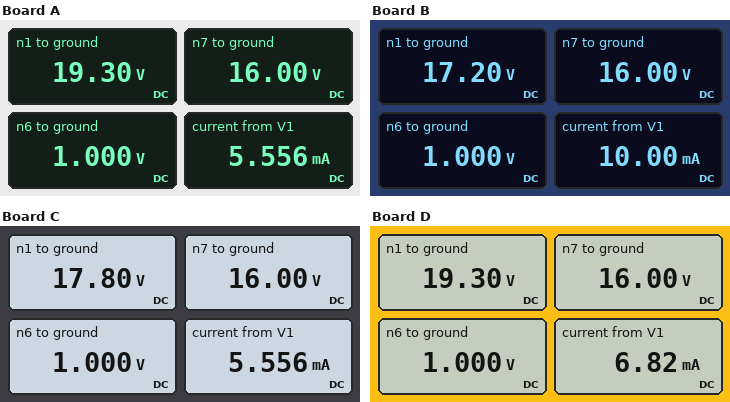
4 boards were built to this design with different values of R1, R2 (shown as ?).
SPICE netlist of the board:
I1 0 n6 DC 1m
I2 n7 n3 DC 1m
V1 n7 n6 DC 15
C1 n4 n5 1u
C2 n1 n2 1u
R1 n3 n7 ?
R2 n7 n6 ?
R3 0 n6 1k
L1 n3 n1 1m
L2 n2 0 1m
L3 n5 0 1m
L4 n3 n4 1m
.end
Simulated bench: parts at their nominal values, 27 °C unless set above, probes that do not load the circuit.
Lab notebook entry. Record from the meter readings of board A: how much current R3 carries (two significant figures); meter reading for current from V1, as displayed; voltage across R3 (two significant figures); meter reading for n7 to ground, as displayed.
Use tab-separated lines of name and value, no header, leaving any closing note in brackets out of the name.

how much current R3 carries	1.0 mA
meter reading for current from V1, as displayed	5.556 mA
voltage across R3	1.0 V
meter reading for n7 to ground, as displayed	16.00 V
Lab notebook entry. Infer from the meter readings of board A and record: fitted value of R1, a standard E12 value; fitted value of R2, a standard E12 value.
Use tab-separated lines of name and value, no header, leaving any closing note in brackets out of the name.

fitted value of R1, a standard E12 value	3.3 kΩ
fitted value of R2, a standard E12 value	2.7 kΩ
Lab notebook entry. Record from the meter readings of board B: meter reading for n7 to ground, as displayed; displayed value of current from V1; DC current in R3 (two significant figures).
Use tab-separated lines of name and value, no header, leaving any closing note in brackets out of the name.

meter reading for n7 to ground, as displayed	16.00 V
displayed value of current from V1	10.00 mA
DC current in R3	1.0 mA
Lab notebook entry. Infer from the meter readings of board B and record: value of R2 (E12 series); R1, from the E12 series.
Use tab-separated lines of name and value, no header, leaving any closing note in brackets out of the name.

value of R2	1.5 kΩ
R1, from the E12 series	1.2 kΩ
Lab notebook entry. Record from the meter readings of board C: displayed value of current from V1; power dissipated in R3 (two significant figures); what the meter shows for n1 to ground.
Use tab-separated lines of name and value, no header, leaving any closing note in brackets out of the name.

displayed value of current from V1	5.556 mA
power dissipated in R3	1.0 mW
what the meter shows for n1 to ground	17.80 V
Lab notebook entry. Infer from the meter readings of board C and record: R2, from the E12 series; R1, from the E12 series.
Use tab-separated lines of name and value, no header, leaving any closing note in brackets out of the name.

R2, from the E12 series	2.7 kΩ
R1, from the E12 series	1.8 kΩ
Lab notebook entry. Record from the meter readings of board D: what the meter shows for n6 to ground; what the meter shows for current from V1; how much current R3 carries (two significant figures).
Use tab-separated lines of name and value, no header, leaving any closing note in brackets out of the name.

what the meter shows for n6 to ground	1.000 V
what the meter shows for current from V1	6.82 mA
how much current R3 carries	1.0 mA
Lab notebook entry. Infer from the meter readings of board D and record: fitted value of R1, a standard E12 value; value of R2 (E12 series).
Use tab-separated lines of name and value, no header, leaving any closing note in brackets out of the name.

fitted value of R1, a standard E12 value	3.3 kΩ
value of R2	2.2 kΩ
